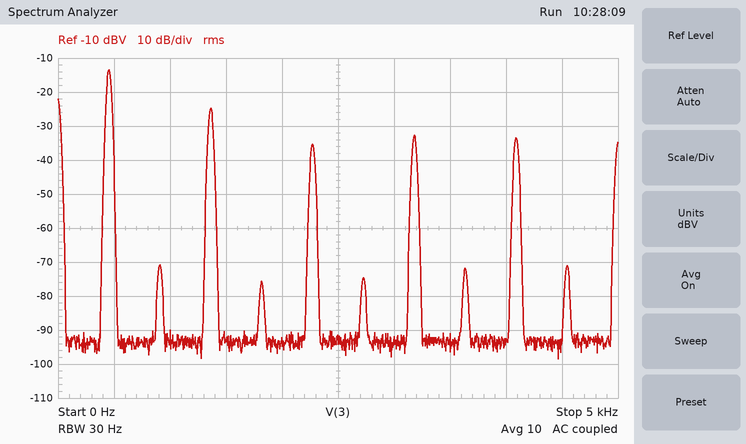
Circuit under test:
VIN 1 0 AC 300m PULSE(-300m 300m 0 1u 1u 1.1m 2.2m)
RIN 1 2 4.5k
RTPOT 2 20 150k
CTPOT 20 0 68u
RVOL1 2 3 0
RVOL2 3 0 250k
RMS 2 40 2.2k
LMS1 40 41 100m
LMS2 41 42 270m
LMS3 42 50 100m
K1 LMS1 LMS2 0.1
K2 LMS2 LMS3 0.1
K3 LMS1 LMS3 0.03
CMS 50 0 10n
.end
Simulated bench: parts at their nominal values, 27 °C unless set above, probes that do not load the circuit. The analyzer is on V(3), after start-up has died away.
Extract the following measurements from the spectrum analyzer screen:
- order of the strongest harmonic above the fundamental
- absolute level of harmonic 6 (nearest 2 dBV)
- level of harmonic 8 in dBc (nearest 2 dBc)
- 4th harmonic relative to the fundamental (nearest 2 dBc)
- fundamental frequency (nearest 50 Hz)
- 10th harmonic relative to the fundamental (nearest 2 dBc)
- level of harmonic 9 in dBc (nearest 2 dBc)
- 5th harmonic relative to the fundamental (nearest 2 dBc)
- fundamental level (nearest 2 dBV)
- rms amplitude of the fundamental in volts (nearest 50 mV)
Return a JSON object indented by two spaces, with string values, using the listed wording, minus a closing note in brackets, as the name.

{
  "order of the strongest harmonic above the fundamental": "3",
  "absolute level of harmonic 6": "-74 dBV",
  "level of harmonic 8 in dBc": "-58 dBc",
  "4th harmonic relative to the fundamental": "-62 dBc",
  "fundamental frequency": "450 Hz",
  "10th harmonic relative to the fundamental": "-58 dBc",
  "level of harmonic 9 in dBc": "-20 dBc",
  "5th harmonic relative to the fundamental": "-22 dBc",
  "fundamental level": "-14 dBV",
  "rms amplitude of the fundamental in volts": "200 mV"
}
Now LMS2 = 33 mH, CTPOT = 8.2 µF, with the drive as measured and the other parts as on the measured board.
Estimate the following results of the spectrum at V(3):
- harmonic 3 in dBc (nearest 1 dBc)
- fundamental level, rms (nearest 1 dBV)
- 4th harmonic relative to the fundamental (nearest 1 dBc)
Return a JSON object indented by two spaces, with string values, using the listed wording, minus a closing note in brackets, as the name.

{
  "harmonic 3 in dBc": "-11 dBc",
  "fundamental level, rms": "-13 dBV",
  "4th harmonic relative to the fundamental": "-59 dBc"
}
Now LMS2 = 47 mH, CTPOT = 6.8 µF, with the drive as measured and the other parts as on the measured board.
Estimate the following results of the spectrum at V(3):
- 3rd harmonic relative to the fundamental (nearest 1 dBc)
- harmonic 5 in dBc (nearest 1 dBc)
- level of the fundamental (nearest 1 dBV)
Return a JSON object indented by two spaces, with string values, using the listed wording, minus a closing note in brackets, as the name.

{
  "3rd harmonic relative to the fundamental": "-11 dBc",
  "harmonic 5 in dBc": "-19 dBc",
  "level of the fundamental": "-13 dBV"
}
